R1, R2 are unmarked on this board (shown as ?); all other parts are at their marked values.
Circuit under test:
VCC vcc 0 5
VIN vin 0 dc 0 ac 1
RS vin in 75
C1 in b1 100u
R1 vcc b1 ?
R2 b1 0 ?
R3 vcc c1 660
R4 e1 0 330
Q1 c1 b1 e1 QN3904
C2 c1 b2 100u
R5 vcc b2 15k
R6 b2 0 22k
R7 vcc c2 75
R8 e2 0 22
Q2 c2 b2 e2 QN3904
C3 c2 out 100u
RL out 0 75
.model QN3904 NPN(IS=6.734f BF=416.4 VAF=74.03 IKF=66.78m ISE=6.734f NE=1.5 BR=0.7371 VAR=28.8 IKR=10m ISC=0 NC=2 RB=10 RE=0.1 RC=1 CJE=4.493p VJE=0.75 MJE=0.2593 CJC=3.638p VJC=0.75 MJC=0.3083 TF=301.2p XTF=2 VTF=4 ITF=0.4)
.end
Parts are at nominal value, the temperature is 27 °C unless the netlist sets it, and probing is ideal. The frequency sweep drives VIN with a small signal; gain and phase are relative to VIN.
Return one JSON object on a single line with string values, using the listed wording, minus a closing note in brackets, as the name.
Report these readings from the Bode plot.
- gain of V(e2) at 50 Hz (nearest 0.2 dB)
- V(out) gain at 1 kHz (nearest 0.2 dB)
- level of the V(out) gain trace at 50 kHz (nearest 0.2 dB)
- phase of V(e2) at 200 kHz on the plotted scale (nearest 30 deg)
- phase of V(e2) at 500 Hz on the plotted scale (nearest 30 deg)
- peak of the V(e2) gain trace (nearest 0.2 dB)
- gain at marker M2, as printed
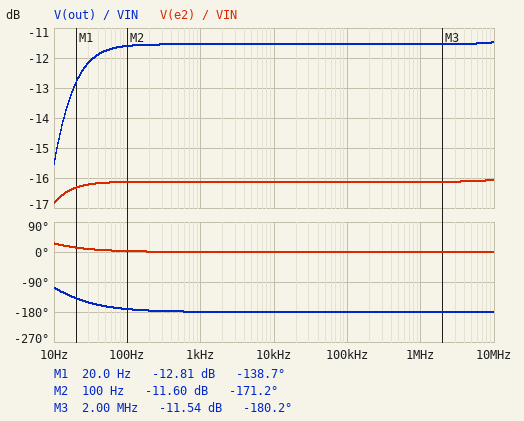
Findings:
{"gain of V(e2) at 50 Hz": "-16.2 dB", "V(out) gain at 1 kHz": "-11.6 dB", "level of the V(out) gain trace at 50 kHz": "-11.6 dB", "phase of V(e2) at 200 kHz on the plotted scale": "0 deg", "phase of V(e2) at 500 Hz on the plotted scale": "0 deg", "peak of the V(e2) gain trace": "-16.0 dB", "gain at marker M2, as printed": "-11.60 dB"}
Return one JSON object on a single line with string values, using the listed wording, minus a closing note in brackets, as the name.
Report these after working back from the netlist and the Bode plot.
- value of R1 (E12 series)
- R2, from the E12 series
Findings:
{"value of R1": "18 kΩ", "R2, from the E12 series": "100 kΩ"}
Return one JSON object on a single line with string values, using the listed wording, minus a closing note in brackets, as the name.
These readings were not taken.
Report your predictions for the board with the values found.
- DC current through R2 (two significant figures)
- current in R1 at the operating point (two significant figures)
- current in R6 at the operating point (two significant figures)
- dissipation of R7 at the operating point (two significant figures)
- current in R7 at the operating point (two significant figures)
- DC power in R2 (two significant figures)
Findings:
{"DC current through R2": "24 µA", "current in R1 at the operating point": "150 µA", "current in R6 at the operating point": "74 µA", "dissipation of R7 at the operating point": "110 mW", "current in R7 at the operating point": "38 mA", "DC power in R2": "56 µW"}
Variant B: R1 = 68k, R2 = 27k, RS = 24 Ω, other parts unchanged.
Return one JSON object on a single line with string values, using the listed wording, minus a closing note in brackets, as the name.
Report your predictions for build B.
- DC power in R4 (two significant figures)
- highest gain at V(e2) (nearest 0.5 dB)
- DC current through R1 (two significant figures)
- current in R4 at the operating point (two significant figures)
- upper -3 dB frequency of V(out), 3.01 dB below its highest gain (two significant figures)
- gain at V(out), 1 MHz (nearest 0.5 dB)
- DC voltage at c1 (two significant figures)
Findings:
{"DC power in R4": "1.2 mW", "highest gain at V(e2)": "3.5 dB", "DC current through R1": "54 µA", "current in R4 at the operating point": "1.9 mA", "upper -3 dB frequency of V(out), 3.01 dB below its highest gain": "11 MHz", "gain at V(out), 1 MHz": "8.0 dB", "DC voltage at c1": "3.7 V"}
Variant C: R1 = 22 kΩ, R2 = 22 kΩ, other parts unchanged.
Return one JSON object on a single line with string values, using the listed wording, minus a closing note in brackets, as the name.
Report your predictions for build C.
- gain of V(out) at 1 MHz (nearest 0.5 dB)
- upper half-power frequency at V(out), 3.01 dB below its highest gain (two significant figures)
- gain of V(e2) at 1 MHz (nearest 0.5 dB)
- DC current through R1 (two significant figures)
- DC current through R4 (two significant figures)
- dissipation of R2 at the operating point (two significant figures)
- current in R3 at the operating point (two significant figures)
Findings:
{"gain of V(out) at 1 MHz": "7.0 dB", "upper half-power frequency at V(out), 3.01 dB below its highest gain": "11 MHz", "gain of V(e2) at 1 MHz": "2.0 dB", "DC current through R1": "120 µA", "DC current through R4": "4.9 mA", "dissipation of R2 at the operating point": "240 µW", "current in R3 at the operating point": "4.8 mA"}
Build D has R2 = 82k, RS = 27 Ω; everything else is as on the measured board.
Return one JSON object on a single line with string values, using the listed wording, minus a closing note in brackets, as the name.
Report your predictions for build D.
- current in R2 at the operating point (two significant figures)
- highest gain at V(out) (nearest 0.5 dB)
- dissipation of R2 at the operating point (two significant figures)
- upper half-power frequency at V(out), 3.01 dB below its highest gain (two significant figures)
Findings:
{"current in R2 at the operating point": "29 µA", "highest gain at V(out)": "-10.0 dB", "dissipation of R2 at the operating point": "68 µW", "upper half-power frequency at V(out), 3.01 dB below its highest gain": "820 MHz"}
